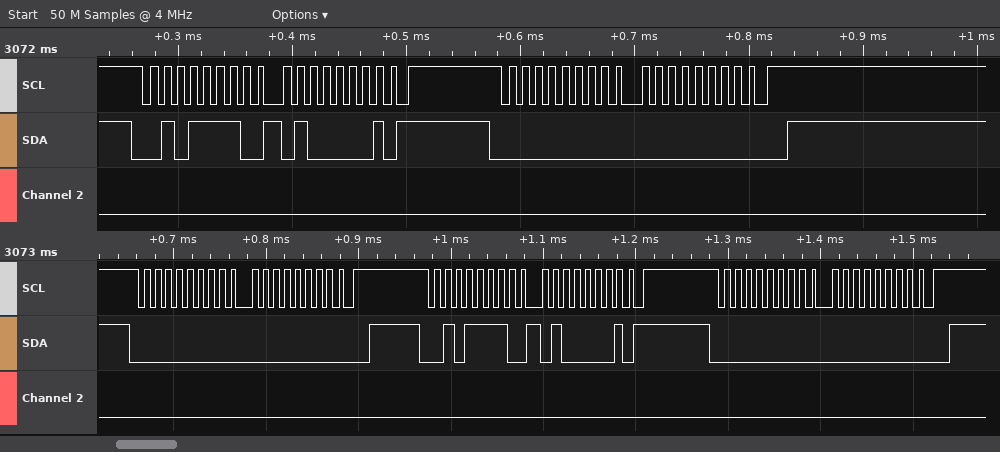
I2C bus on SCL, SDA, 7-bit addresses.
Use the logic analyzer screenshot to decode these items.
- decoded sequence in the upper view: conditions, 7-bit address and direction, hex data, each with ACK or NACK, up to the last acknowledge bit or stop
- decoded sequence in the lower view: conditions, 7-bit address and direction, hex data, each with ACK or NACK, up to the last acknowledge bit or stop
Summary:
start, address 2F write ACK, 41 ACK, repeated start, address 00 write ACK, 00 ACK, stop
start, address 00 write ACK, 00 ACK, stop, start, address 2F write ACK, 41 ACK, repeated start, address 00 write ACK, 00 ACK, stop
